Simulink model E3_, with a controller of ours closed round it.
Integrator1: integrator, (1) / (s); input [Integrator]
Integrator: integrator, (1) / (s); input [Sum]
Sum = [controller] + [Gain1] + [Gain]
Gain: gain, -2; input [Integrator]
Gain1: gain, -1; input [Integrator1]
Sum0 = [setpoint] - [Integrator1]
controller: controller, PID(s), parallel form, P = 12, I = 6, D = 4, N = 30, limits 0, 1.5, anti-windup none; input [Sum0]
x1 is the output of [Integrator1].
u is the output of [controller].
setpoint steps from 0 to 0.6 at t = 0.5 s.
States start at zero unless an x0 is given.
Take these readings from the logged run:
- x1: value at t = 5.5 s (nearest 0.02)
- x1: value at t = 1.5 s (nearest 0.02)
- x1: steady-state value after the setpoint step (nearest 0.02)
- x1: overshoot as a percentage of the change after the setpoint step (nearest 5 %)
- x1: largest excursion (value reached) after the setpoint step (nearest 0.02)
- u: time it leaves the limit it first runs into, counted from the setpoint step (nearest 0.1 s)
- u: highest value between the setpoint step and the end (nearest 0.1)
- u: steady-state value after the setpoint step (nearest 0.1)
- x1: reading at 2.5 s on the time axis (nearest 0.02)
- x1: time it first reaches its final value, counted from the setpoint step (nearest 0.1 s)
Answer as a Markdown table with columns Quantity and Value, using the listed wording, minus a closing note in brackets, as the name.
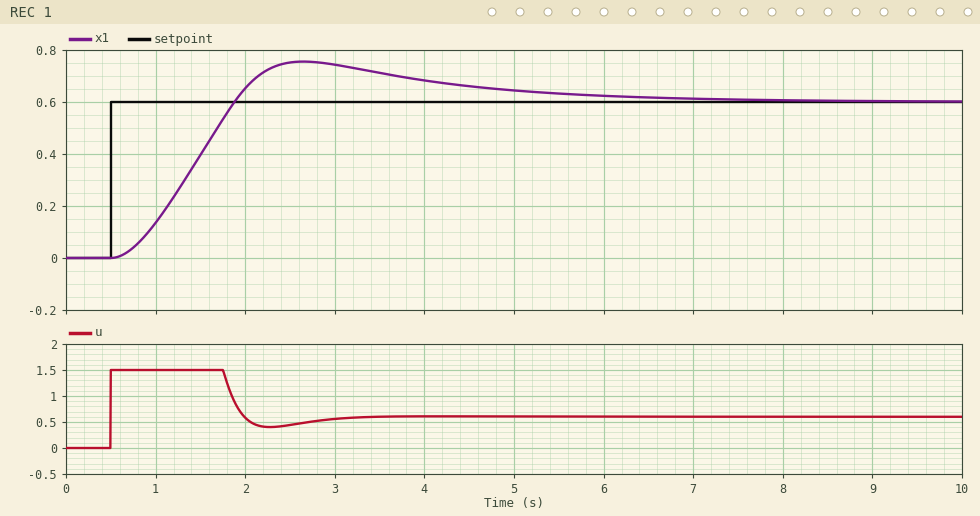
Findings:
| Quantity | Value |
|---|---|
| x1: value at t = 5.5 s | 0.64 |
| x1: value at t = 1.5 s | 0.40 |
| x1: steady-state value after the setpoint step | 0.60 |
| x1: overshoot as a percentage of the change after the setpoint step | 25 % |
| x1: largest excursion (value reached) after the setpoint step | 0.76 |
| u: time it leaves the limit it first runs into, counted from the setpoint step | 1.3 s |
| u: highest value between the setpoint step and the end | 1.5 |
| u: steady-state value after the setpoint step | 0.6 |
| x1: reading at 2.5 s on the time axis | 0.76 |
| x1: time it first reaches its final value, counted from the setpoint step | 1.4 s |
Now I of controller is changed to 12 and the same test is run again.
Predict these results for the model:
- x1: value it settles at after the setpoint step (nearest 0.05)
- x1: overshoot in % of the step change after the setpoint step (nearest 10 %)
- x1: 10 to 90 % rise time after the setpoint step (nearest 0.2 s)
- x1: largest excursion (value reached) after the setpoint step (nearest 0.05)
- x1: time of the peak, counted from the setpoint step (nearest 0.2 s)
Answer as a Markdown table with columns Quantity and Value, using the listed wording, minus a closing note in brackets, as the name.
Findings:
| Quantity | Value |
|---|---|
| x1: value it settles at after the setpoint step | 0.60 |
| x1: overshoot in % of the step change after the setpoint step | 50 % |
| x1: 10 to 90 % rise time after the setpoint step | 1.0 s |
| x1: largest excursion (value reached) after the setpoint step | 0.90 |
| x1: time of the peak, counted from the setpoint step | 2.2 s |
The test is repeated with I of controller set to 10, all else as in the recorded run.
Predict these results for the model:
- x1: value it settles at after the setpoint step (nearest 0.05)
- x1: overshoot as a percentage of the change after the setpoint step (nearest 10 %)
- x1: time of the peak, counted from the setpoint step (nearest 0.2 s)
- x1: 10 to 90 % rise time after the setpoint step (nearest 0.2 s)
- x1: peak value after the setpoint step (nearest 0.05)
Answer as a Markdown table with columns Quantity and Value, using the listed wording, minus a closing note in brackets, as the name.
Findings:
| Quantity | Value |
|---|---|
| x1: value it settles at after the setpoint step | 0.60 |
| x1: overshoot as a percentage of the change after the setpoint step | 40 % |
| x1: time of the peak, counted from the setpoint step | 2.2 s |
| x1: 10 to 90 % rise time after the setpoint step | 1.0 s |
| x1: peak value after the setpoint step | 0.85 |
